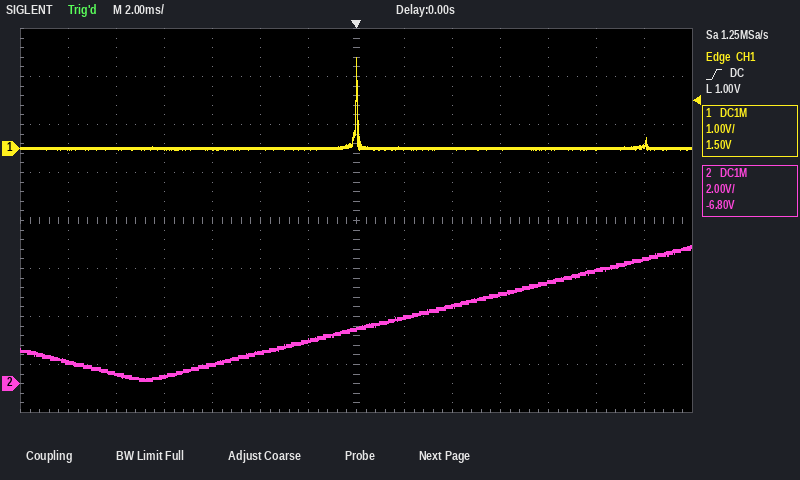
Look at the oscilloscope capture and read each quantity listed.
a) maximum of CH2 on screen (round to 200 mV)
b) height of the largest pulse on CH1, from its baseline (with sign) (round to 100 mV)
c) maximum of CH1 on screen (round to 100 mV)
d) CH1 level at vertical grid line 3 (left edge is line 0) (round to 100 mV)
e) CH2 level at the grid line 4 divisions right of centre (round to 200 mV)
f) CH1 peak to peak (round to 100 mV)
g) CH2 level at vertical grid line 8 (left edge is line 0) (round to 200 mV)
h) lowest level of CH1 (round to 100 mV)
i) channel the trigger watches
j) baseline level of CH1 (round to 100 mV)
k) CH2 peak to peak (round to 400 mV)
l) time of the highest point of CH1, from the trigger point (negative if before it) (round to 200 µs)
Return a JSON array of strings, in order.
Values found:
["5.8 V", "+1.9 V", "1.9 V", "0.0 V", "4.2 V", "1.9 V", "2.8 V", "0.0 V", "CH1", "0.0 V", "5.6 V", "0.0 ms"]
